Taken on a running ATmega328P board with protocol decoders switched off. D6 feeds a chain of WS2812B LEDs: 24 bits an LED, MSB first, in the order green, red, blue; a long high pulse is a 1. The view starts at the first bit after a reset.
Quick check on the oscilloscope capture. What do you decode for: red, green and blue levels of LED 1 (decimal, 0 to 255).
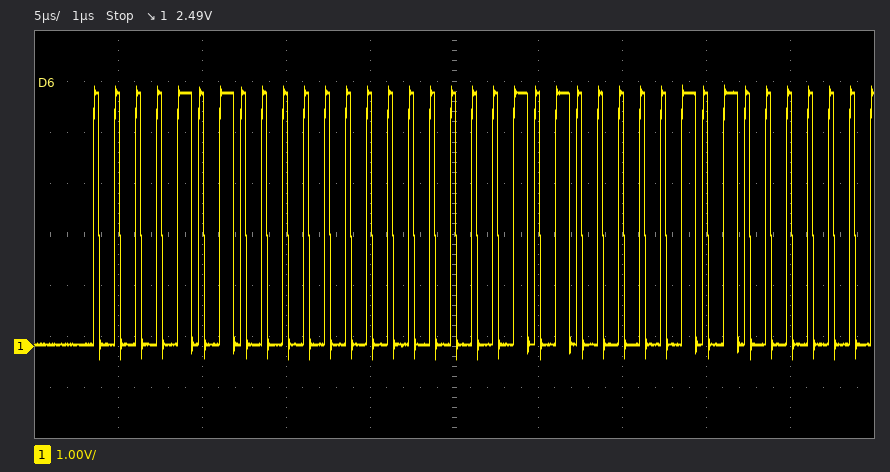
0, 10, 10
